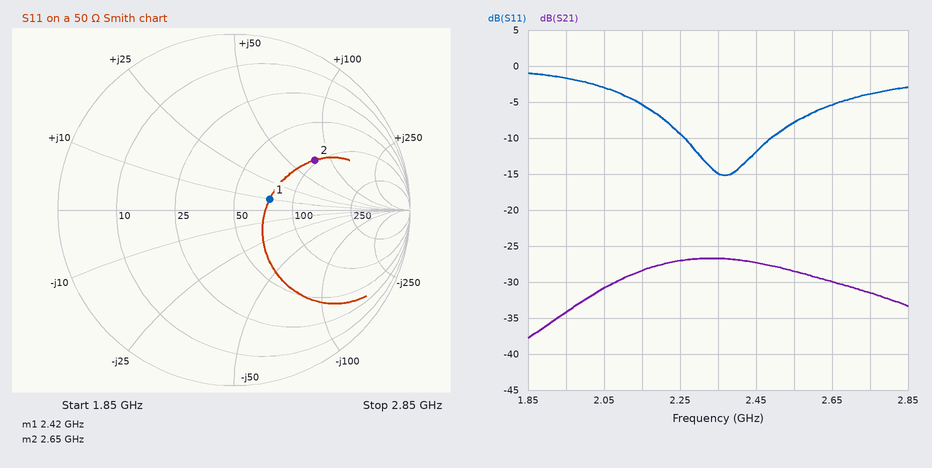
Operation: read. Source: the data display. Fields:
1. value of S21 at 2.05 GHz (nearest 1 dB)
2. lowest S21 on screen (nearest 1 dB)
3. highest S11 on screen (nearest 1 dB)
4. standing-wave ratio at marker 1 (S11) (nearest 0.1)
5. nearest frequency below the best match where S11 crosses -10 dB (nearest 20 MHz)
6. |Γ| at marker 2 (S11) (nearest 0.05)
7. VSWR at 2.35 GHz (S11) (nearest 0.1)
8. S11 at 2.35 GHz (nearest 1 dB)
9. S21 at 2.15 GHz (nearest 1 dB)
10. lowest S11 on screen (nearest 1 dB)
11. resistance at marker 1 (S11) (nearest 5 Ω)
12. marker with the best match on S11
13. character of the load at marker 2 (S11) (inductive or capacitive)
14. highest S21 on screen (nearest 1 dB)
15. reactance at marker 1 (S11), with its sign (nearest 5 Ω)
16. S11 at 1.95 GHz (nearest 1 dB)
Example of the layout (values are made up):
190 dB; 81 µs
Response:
-31 dB; -38 dB; -1 dB; 1.5; 2.26 GHz; 0.55; 1.4; -15 dB; -28 dB; -15 dB; 75 Ω; marker 1; inductive; -27 dB; +10 Ω; -2 dB
